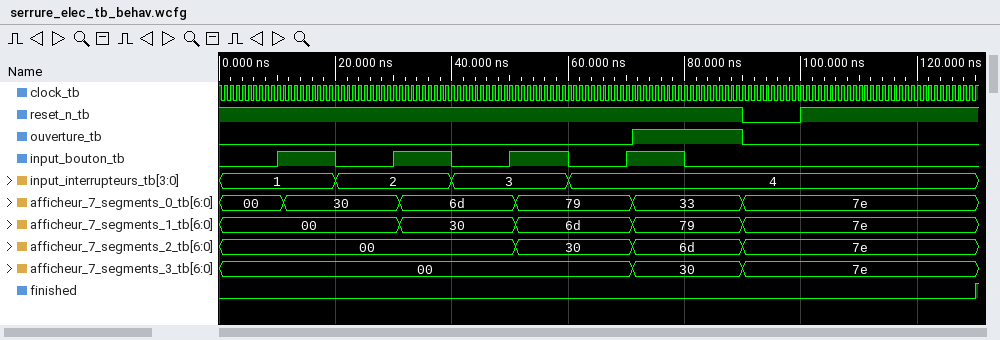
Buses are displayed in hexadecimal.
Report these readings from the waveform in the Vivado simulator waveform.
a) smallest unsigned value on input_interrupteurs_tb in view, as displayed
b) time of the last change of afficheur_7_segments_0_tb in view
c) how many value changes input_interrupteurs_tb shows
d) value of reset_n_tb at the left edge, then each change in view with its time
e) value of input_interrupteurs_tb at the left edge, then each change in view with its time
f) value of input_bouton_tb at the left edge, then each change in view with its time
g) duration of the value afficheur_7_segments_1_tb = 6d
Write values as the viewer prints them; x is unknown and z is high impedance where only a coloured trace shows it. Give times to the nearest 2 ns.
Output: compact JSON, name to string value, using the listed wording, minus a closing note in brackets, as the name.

{"smallest unsigned value on input_interrupteurs_tb in view, as displayed": "1", "time of the last change of afficheur_7_segments_0_tb in view": "90 ns", "how many value changes input_interrupteurs_tb shows": "3", "value of reset_n_tb at the left edge, then each change in view with its time": "1, 0 at 90 ns, 1 at 100 ns", "value of input_interrupteurs_tb at the left edge, then each change in view with its time": "1, 2 at 20 ns, 3 at 40 ns, 4 at 60 ns", "value of input_bouton_tb at the left edge, then each change in view with its time": "0, 1 at 10 ns, 0 at 20 ns, 1 at 30 ns, 0 at 40 ns, 1 at 50 ns, 0 at 60 ns, 1 at 70 ns, 0 at 80 ns", "duration of the value afficheur_7_segments_1_tb = 6d": "20 ns"}
